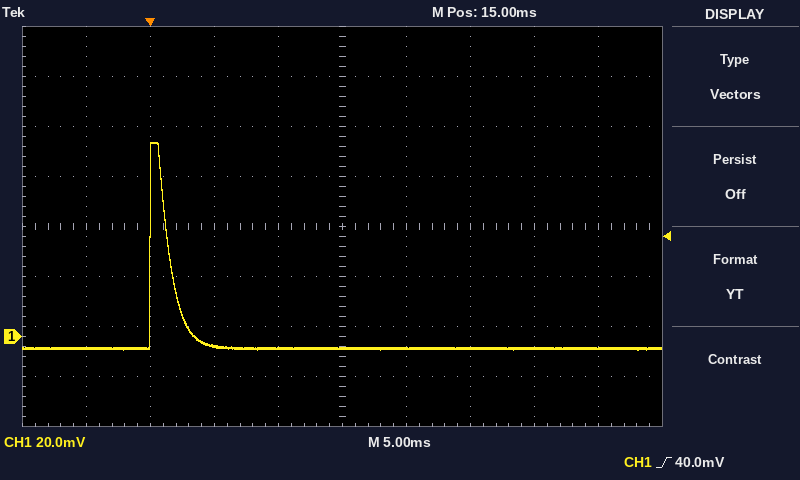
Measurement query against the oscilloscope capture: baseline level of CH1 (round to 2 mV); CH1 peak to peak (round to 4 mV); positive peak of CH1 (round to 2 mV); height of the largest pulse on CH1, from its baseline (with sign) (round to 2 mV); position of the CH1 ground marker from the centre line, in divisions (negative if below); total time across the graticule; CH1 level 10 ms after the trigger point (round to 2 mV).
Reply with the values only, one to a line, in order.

-4 mV
84 mV
78 mV
+82 mV
-2.2 div
50 ms
-4 mV
